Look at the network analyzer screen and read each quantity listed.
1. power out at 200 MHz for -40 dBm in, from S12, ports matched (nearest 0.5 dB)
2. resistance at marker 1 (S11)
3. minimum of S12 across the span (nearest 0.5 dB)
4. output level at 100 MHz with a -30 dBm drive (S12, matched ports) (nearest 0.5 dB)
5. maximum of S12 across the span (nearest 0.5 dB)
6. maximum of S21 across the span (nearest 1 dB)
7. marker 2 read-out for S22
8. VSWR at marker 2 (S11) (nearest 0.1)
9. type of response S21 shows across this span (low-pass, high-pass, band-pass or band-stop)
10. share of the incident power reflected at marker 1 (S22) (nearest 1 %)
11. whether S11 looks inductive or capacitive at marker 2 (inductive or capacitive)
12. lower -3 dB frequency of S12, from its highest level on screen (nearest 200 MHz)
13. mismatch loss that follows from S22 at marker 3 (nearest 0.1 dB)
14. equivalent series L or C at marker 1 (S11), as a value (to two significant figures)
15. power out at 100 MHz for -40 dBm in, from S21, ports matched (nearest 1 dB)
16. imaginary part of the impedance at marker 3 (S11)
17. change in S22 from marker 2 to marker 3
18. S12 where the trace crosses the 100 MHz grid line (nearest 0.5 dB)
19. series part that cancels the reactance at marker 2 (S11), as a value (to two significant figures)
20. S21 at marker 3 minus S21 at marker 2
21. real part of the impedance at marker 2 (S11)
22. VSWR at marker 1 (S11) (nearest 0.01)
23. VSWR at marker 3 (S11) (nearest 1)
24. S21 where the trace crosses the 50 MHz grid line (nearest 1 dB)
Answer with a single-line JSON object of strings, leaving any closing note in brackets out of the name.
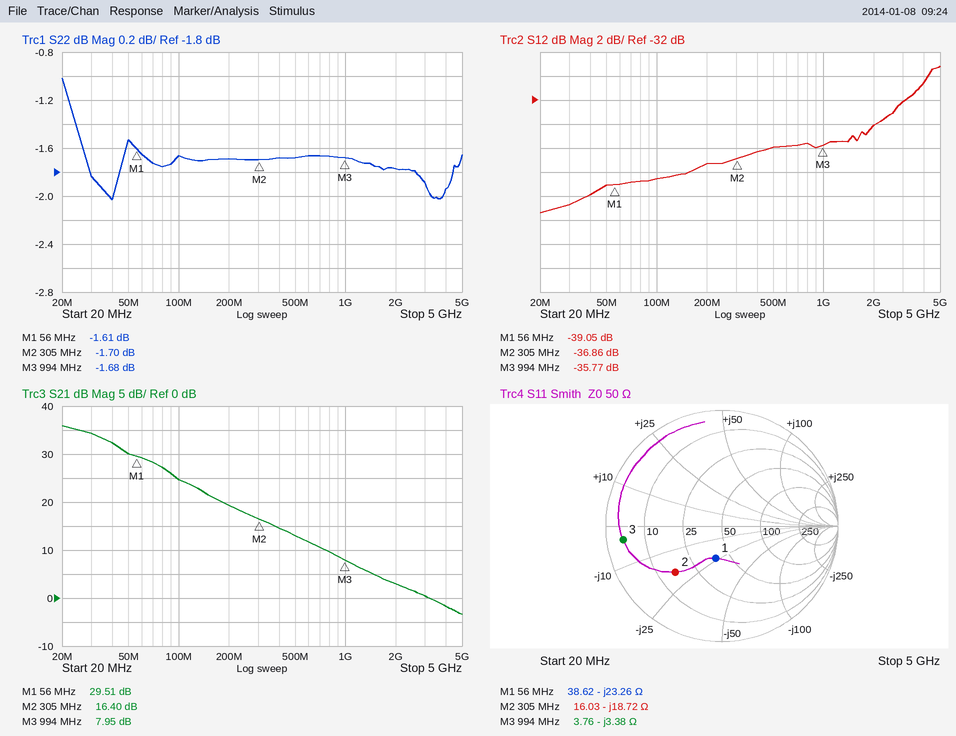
{"power out at 200 MHz for -40 dBm in, from S12, ports matched": "-77.5 dBm", "resistance at marker 1": "38.62 Ω", "minimum of S12 across the span": "-41.5 dB", "output level at 100 MHz with a -30 dBm drive (S12, matched ports)": "-68.5 dBm", "maximum of S12 across the span": "-29.0 dB", "maximum of S21 across the span": "36 dB", "marker 2 read-out for S22": "-1.70 dB", "VSWR at marker 2 (S11)": "3.6", "type of response S21 shows across this span": "low-pass", "share of the incident power reflected at marker 1 (S22)": "69 %", "whether S11 looks inductive or capacitive at marker 2": "capacitive", "lower -3 dB frequency of S12, from its highest level on screen": "3.0 GHz", "mismatch loss that follows from S22 at marker 3": "4.9 dB", "equivalent series L or C at marker 1 (S11), as a value": "120 pF", "power out at 100 MHz for -40 dBm in, from S21, ports matched": "-15 dBm", "imaginary part of the impedance at marker 3": "-3.38 Ω", "change in S22 from marker 2 to marker 3": "0.02 dB", "S12 where the trace crosses the 100 MHz grid line": "-38.5 dB", "series part that cancels the reactance at marker 2 (S11), as a value": "9.8 nH", "S21 at marker 3 minus S21 at marker 2": "-8.45 dB", "real part of the impedance at marker 2": "16.03 Ω", "VSWR at marker 1 (S11)": "1.79", "VSWR at marker 3 (S11)": "13", "S21 where the trace crosses the 50 MHz grid line": "30 dB"}
